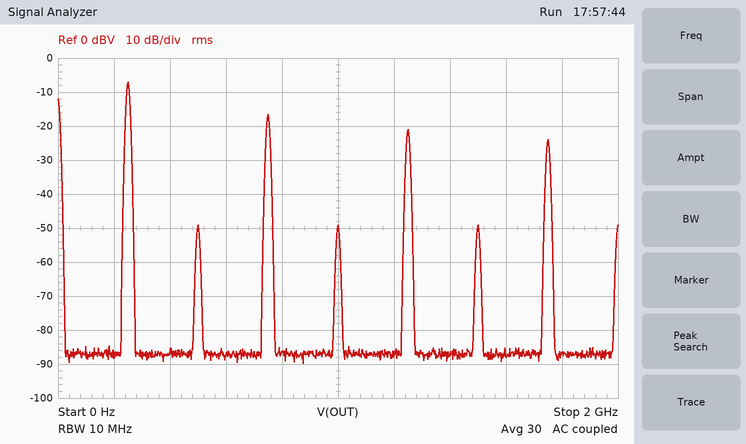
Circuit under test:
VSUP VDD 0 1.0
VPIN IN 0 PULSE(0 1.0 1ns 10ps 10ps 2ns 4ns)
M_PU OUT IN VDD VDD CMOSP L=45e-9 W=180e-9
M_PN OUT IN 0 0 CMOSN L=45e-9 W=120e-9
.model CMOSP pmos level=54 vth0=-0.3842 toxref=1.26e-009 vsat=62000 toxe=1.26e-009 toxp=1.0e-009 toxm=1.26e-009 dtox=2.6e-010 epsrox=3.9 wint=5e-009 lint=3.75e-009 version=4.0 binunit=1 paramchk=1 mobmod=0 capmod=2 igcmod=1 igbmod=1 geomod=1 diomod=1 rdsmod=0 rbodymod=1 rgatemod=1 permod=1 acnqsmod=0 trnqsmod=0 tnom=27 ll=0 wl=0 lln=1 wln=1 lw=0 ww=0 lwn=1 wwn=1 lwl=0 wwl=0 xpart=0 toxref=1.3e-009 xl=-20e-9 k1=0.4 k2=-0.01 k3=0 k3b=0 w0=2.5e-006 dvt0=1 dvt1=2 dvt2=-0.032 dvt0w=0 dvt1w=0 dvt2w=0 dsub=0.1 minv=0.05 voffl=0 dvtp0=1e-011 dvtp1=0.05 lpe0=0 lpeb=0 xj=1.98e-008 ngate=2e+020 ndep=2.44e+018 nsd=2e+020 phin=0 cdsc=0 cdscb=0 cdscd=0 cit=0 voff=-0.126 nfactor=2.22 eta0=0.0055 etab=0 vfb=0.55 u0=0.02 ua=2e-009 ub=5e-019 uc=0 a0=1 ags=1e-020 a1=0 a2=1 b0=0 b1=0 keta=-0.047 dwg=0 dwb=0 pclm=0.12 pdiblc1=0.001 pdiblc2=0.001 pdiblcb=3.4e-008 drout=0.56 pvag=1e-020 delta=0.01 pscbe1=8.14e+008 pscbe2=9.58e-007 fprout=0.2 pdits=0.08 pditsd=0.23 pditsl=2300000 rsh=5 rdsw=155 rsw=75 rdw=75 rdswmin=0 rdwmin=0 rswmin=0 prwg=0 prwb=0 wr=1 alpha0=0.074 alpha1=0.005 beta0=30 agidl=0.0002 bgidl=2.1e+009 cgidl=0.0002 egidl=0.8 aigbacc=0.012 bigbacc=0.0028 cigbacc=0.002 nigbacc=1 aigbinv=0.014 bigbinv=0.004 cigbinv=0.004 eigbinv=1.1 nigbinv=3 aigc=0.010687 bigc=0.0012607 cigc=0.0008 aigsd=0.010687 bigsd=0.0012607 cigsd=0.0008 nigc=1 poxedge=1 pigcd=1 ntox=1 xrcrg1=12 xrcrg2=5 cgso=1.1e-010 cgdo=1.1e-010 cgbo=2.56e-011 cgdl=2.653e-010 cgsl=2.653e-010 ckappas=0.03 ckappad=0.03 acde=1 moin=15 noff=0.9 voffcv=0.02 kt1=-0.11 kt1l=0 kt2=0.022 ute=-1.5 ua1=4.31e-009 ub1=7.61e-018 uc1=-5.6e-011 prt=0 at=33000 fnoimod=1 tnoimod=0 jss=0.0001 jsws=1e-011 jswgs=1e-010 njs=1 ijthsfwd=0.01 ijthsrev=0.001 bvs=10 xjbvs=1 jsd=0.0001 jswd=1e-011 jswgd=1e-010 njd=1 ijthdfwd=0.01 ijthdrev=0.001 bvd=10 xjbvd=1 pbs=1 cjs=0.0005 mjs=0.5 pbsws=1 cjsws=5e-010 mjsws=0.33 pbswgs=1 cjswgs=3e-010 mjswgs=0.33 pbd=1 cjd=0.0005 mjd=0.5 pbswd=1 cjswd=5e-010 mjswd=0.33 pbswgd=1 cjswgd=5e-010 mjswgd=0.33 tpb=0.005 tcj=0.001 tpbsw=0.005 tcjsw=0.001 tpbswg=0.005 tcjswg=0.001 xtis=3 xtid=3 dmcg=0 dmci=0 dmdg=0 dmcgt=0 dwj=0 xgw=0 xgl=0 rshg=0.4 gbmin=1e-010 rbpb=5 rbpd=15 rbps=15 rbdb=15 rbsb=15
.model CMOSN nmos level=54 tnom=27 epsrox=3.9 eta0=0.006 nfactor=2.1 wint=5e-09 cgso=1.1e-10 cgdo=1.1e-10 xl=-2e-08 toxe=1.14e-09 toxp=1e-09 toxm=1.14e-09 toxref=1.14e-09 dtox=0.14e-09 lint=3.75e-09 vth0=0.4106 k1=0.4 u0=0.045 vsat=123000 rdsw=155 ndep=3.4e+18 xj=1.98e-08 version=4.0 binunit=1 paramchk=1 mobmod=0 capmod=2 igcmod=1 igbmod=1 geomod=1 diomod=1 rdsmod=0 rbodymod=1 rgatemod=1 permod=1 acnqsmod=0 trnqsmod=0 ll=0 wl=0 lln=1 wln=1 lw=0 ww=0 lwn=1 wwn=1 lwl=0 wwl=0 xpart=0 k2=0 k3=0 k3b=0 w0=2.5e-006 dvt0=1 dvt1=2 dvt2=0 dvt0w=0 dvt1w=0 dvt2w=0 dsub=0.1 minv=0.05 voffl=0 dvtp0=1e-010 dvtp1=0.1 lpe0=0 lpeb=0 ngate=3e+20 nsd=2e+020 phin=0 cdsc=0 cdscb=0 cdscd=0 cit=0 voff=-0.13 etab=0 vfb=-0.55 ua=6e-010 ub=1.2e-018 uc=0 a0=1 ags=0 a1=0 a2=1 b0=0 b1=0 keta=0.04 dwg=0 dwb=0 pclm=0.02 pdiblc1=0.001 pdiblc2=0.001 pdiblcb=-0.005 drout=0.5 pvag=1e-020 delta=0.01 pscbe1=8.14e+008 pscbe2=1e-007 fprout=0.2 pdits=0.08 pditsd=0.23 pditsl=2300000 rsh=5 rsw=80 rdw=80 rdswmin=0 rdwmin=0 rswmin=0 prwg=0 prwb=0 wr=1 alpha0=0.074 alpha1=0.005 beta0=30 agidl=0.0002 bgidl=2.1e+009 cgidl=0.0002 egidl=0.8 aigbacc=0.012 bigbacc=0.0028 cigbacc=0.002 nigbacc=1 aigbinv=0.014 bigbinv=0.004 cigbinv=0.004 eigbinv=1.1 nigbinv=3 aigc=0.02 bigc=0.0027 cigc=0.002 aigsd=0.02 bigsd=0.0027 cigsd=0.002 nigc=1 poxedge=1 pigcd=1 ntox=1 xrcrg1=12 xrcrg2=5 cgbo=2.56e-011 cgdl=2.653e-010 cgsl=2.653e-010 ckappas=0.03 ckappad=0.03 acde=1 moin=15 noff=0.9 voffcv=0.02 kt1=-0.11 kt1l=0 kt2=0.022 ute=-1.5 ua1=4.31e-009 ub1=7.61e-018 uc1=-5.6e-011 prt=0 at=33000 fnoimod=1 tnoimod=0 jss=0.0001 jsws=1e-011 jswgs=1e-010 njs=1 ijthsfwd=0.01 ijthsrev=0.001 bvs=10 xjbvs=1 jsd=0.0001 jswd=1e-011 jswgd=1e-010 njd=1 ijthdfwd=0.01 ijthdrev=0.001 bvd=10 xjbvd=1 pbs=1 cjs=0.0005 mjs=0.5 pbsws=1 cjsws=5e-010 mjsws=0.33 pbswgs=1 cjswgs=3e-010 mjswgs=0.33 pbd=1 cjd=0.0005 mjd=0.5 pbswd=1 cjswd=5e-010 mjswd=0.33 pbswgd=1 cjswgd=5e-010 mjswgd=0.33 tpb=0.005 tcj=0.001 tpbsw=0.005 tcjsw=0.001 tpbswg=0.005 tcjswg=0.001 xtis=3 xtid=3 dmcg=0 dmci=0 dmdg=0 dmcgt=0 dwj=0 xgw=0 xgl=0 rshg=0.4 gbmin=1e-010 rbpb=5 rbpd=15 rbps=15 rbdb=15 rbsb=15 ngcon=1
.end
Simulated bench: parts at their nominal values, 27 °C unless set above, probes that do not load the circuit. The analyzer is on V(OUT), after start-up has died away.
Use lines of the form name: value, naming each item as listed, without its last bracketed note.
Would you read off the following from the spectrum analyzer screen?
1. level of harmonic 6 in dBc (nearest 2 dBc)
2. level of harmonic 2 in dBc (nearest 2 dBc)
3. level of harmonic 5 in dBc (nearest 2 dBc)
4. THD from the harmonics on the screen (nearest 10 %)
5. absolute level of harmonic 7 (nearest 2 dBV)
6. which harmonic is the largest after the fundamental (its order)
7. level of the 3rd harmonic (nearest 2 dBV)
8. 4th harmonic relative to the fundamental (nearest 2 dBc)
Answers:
level of harmonic 6 in dBc: -42 dBc
level of harmonic 2 in dBc: -42 dBc
level of harmonic 5 in dBc: -14 dBc
THD from the harmonics on the screen: 40 %
absolute level of harmonic 7: -24 dBV
which harmonic is the largest after the fundamental: 3
level of the 3rd harmonic: -16 dBV
4th harmonic relative to the fundamental: -42 dBc
